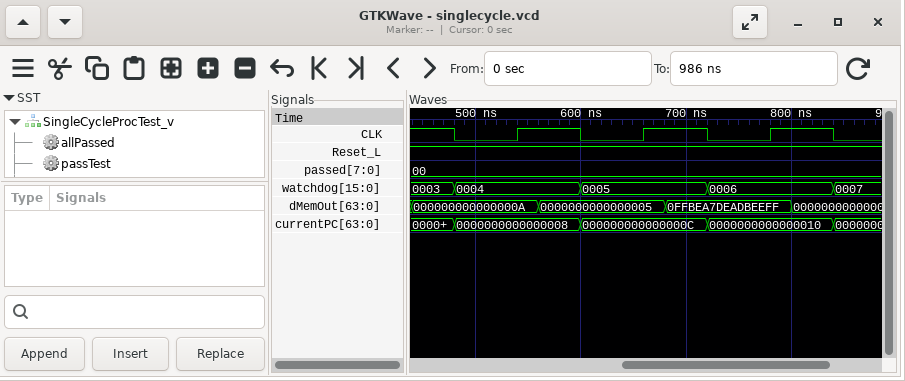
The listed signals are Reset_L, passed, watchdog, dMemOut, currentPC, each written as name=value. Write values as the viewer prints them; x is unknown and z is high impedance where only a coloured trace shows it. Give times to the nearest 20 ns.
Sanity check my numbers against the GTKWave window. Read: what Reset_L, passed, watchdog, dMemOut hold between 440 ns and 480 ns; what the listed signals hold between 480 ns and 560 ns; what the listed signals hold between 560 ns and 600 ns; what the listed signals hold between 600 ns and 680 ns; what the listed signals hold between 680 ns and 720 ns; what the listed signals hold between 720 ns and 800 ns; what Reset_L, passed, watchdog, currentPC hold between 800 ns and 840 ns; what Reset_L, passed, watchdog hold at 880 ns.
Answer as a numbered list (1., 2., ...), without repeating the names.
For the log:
1. Reset_L=1, passed=00, watchdog=0003, dMemOut=000000000000000A
2. Reset_L=1, passed=00, watchdog=0004, dMemOut=000000000000000A, currentPC=0000000000000008
3. Reset_L=1, passed=00, watchdog=0004, dMemOut=0000000000000005, currentPC=0000000000000008
4. Reset_L=1, passed=00, watchdog=0005, dMemOut=0000000000000005, currentPC=000000000000000C
5. Reset_L=1, passed=00, watchdog=0005, dMemOut=0FFBEA7DEADBEEFF, currentPC=000000000000000C
6. Reset_L=1, passed=00, watchdog=0006, dMemOut=0FFBEA7DEADBEEFF, currentPC=0000000000000010
7. Reset_L=1, passed=00, watchdog=0006, currentPC=0000000000000010
8. Reset_L=1, passed=00, watchdog=0007
